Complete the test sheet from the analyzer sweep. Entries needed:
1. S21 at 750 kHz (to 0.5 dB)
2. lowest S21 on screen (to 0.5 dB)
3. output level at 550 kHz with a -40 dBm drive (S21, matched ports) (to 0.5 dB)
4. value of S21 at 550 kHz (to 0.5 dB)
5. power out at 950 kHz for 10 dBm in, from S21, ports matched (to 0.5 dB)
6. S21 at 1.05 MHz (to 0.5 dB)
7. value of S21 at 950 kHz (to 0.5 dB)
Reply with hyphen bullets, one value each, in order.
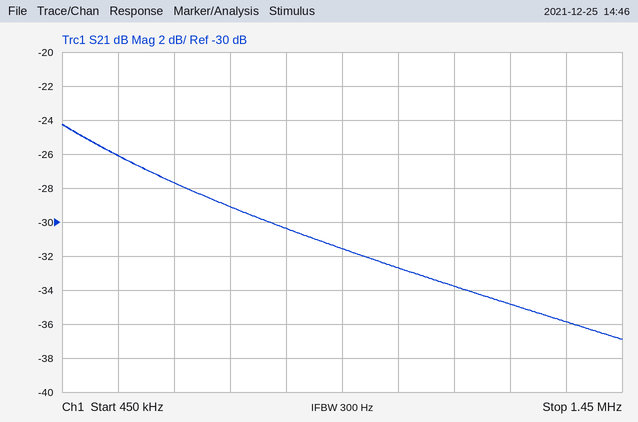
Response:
- -29.0 dB
- -37.0 dB
- -66.0 dBm
- -26.0 dB
- -21.5 dBm
- -32.5 dB
- -31.5 dB
